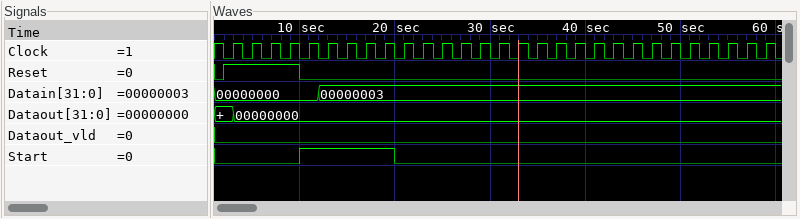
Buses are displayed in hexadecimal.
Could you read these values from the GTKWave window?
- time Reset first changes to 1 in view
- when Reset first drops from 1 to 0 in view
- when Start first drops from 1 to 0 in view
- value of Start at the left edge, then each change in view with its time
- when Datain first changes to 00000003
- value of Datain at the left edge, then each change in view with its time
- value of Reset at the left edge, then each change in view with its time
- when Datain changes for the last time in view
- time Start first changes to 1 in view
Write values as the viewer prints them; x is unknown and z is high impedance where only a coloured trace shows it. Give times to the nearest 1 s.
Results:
2 s
10 s
20 s
0, 1 at 10 s, 0 at 20 s
12 s
00000000, 00000003 at 12 s
0, 1 at 2 s, 0 at 10 s
12 s
10 s
